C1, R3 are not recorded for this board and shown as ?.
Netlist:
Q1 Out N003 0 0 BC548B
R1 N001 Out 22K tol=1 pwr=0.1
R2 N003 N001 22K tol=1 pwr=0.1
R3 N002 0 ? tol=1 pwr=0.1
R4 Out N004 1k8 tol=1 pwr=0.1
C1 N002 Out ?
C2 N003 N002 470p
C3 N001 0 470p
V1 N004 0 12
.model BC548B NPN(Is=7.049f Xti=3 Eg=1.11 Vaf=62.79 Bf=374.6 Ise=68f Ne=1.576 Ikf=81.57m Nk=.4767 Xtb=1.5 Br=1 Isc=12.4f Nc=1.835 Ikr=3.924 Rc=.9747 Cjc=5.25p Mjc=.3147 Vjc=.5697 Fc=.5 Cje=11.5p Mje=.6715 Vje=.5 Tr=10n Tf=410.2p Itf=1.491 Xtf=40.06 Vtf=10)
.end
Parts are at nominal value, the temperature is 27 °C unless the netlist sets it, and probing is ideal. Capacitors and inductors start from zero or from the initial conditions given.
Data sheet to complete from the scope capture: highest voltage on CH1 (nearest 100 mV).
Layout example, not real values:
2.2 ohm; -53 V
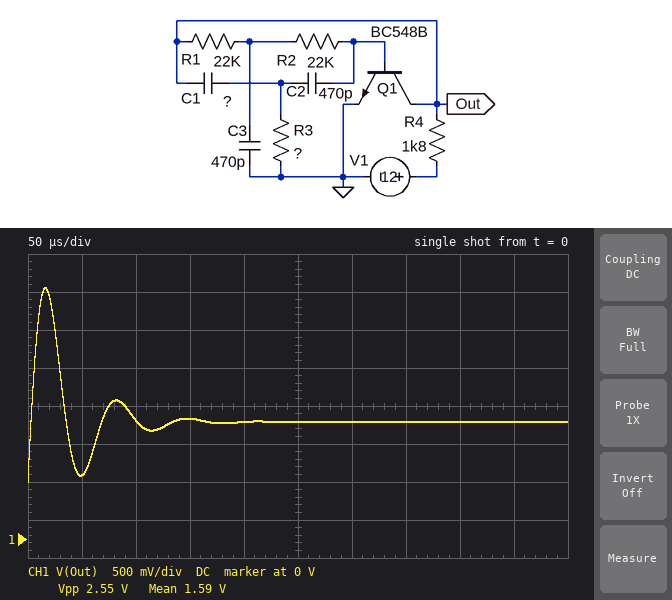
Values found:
3.3 V
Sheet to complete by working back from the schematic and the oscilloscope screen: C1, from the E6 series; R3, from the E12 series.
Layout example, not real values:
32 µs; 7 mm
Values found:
680 pF; 10 kΩ
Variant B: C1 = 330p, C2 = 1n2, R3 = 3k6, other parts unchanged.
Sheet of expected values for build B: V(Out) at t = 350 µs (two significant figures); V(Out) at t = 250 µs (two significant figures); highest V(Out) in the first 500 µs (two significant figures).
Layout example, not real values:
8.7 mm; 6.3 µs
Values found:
1.6 V; 1.7 V; 7.0 V
